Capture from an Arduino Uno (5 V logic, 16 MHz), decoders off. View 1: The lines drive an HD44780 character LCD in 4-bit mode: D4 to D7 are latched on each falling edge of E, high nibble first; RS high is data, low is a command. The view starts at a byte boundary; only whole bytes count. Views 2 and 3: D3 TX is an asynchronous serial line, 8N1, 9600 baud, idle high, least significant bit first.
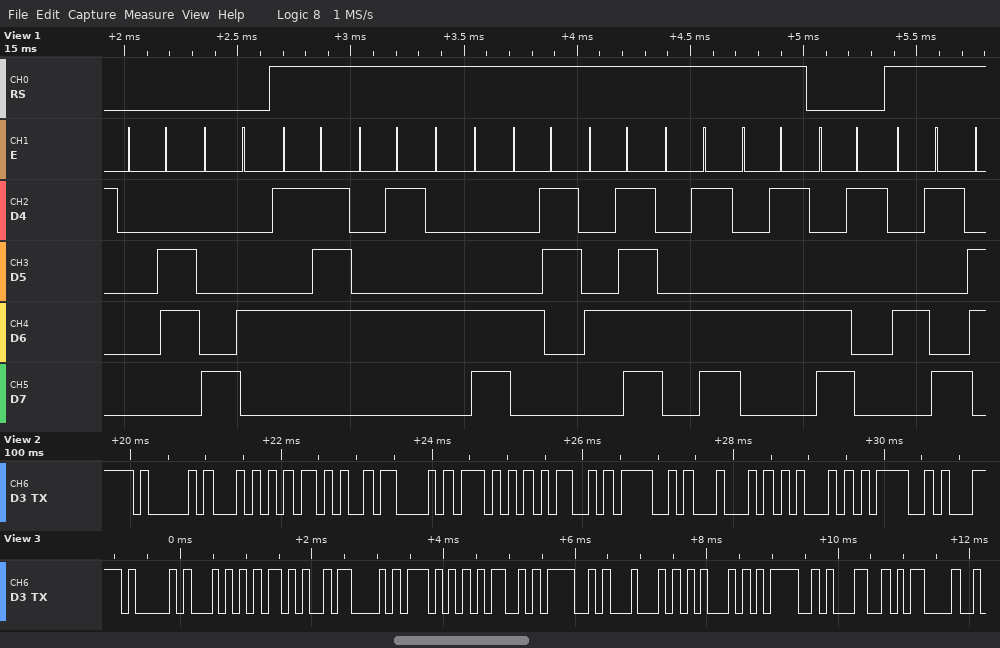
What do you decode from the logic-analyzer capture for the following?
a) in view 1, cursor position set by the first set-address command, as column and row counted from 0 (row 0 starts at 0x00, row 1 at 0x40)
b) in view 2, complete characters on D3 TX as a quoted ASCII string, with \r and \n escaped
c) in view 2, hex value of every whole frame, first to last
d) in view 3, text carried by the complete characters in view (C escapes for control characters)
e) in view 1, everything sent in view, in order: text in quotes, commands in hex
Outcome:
column 4, row 0
"AT+CWMODE="
41 54 2B 43 57 4D 4F 44 45 3D
"AT+CWMODE=1\r"
0x06 0x84 "WELCOME" 0xC1 "I"
